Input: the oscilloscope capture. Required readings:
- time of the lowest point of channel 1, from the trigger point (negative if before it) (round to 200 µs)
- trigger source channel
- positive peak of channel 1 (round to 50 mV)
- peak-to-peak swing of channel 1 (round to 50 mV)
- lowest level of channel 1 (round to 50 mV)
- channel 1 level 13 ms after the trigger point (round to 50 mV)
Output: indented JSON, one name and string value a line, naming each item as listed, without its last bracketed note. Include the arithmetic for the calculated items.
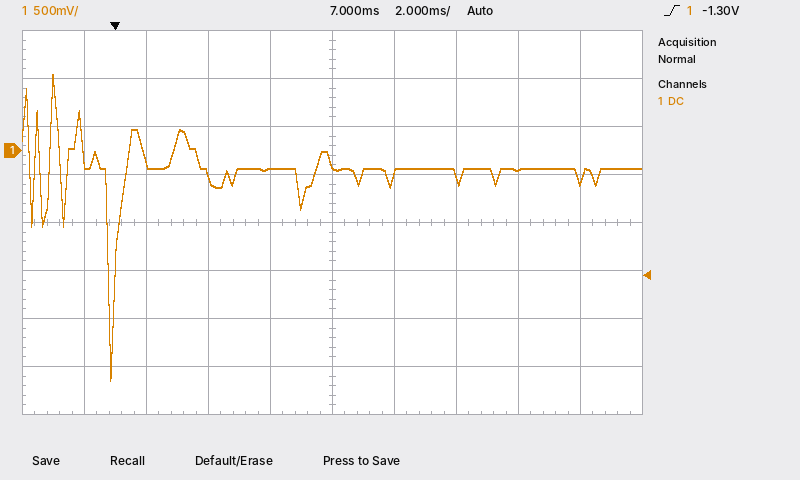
{
  "time of the lowest point of channel 1, from the trigger point (negative if before it)": "-200 µs",
  "trigger source channel": "channel 1",
  "positive peak of channel 1": "800 mV",
  "peak-to-peak swing of channel 1": "800 mV − (-2.40 V) = 3.20 V",
  "lowest level of channel 1": "-2.40 V",
  "channel 1 level 13 ms after the trigger point": "-200 mV"
}
